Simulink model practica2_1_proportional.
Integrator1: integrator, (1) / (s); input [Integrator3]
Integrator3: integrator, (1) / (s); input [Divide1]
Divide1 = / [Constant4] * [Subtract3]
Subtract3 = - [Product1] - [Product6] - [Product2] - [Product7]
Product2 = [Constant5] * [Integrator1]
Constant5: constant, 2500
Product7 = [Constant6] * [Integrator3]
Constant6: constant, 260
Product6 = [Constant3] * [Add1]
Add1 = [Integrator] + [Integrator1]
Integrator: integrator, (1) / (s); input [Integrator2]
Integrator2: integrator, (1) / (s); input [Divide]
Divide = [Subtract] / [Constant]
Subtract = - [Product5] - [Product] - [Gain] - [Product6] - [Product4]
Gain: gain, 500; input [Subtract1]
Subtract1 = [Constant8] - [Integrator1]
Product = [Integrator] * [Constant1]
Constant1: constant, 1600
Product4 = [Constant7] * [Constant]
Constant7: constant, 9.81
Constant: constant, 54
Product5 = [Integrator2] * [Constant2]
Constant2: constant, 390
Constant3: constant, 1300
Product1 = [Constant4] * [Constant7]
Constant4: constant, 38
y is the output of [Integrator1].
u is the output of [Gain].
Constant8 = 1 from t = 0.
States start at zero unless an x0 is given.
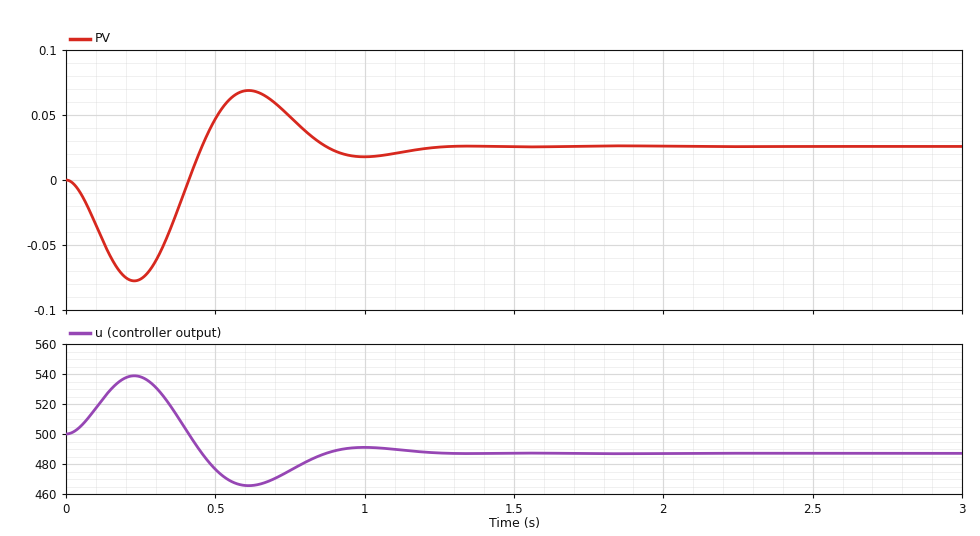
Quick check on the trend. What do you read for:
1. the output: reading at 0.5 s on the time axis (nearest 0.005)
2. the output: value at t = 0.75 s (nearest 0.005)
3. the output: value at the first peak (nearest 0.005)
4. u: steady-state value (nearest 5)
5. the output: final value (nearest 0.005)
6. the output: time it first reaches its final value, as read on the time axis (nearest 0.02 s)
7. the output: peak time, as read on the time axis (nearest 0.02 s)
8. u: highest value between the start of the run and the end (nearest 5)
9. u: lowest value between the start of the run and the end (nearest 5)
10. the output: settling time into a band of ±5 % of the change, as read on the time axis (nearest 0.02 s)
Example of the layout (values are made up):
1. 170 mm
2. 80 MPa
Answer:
1. 0.045
2. 0.050
3. 0.070
4. 485
5. 0.025
6. 0.46 s
7. 0.62 s
8. 540
9. 465
10. 1.22 s
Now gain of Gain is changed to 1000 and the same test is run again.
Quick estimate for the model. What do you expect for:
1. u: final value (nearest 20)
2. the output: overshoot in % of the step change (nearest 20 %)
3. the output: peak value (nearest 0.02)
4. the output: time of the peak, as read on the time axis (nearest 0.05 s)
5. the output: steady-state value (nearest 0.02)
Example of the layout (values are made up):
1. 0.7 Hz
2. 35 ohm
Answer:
1. 920
2. 80 %
3. 0.16
4. 0.60 s
5. 0.08
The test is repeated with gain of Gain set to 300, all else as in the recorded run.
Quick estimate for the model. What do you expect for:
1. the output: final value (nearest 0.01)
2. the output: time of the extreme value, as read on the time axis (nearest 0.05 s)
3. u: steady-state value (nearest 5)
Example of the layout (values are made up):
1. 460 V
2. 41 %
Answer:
1. 0.00
2. 0.25 s
3. 300
